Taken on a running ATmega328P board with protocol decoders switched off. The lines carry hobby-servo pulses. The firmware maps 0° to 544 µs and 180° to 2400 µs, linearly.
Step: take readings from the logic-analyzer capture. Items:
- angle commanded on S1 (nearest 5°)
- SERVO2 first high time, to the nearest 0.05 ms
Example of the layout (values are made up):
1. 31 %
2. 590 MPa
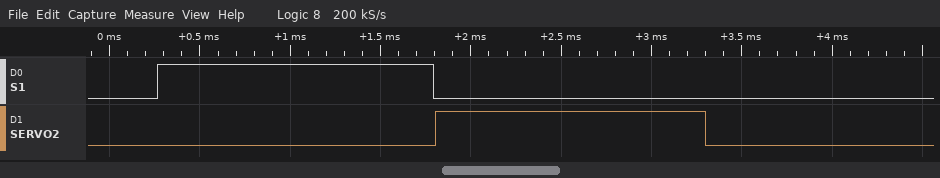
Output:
1. 95°
2. 1.50 ms
